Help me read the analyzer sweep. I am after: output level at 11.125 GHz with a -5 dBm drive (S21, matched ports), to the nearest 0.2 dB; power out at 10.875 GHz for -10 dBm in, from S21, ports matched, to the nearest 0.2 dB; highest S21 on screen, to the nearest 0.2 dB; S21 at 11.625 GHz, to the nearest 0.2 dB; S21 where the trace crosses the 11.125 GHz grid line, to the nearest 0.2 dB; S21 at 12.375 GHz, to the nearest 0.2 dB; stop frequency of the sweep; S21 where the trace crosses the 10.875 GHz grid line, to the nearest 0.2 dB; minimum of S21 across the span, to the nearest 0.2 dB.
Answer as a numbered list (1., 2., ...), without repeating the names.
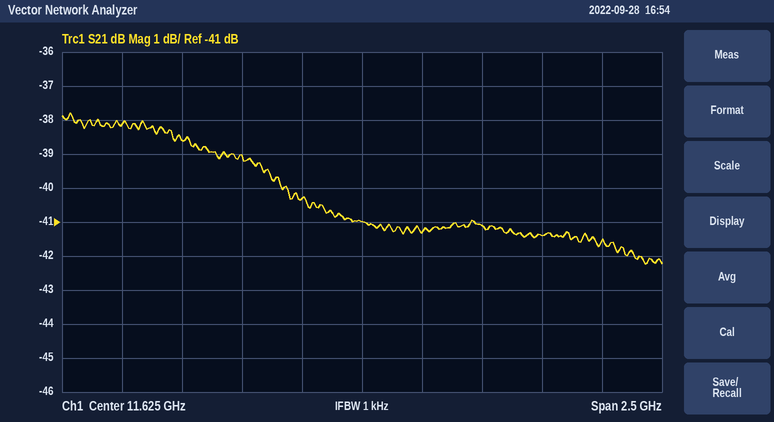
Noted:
1. -44.0 dBm
2. -48.6 dBm
3. -37.8 dB
4. -41.0 dB
5. -39.0 dB
6. -41.4 dB
7. 12.875 GHz
8. -38.6 dB
9. -42.2 dB
